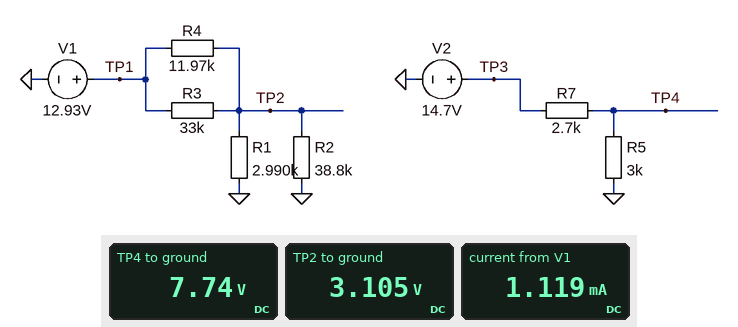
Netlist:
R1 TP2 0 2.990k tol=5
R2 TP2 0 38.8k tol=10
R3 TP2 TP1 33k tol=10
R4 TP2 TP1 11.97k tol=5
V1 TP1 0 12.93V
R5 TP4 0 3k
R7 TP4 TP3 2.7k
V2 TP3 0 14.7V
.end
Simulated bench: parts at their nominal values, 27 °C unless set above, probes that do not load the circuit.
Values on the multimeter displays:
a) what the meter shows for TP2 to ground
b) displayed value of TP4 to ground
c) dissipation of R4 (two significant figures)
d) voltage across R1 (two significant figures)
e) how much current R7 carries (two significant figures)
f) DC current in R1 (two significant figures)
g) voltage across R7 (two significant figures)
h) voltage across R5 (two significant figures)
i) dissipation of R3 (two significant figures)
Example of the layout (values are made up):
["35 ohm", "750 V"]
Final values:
["3.105 V", "7.74 V", "8.1 mW", "3.1 V", "2.6 mA", "1.0 mA", "7.0 V", "7.7 V", "2.9 mW"]
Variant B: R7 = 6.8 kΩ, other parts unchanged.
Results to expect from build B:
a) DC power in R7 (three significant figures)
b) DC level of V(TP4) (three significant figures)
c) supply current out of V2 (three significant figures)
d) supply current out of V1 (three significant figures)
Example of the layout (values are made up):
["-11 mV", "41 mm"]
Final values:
["15.3 mW", "4.50 V", "1.50 mA", "1.12 mA"]
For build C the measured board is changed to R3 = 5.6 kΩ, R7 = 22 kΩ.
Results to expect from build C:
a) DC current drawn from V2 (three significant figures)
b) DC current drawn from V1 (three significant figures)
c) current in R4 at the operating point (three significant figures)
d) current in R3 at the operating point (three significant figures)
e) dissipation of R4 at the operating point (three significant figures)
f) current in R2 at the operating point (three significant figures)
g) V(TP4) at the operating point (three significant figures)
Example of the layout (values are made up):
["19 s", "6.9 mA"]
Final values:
["588 µA", "1.96 mA", "625 µA", "1.34 mA", "4.68 mW", "140 µA", "1.76 V"]
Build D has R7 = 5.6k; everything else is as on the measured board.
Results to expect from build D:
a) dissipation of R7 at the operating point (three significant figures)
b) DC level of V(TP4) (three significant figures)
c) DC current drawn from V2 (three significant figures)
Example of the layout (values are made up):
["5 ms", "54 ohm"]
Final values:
["16.4 mW", "5.13 V", "1.71 mA"]
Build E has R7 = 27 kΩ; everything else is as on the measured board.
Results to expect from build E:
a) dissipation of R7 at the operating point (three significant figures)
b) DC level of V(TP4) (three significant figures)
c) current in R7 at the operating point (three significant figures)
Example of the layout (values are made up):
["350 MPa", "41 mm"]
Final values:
["6.48 mW", "1.47 V", "490 µA"]
